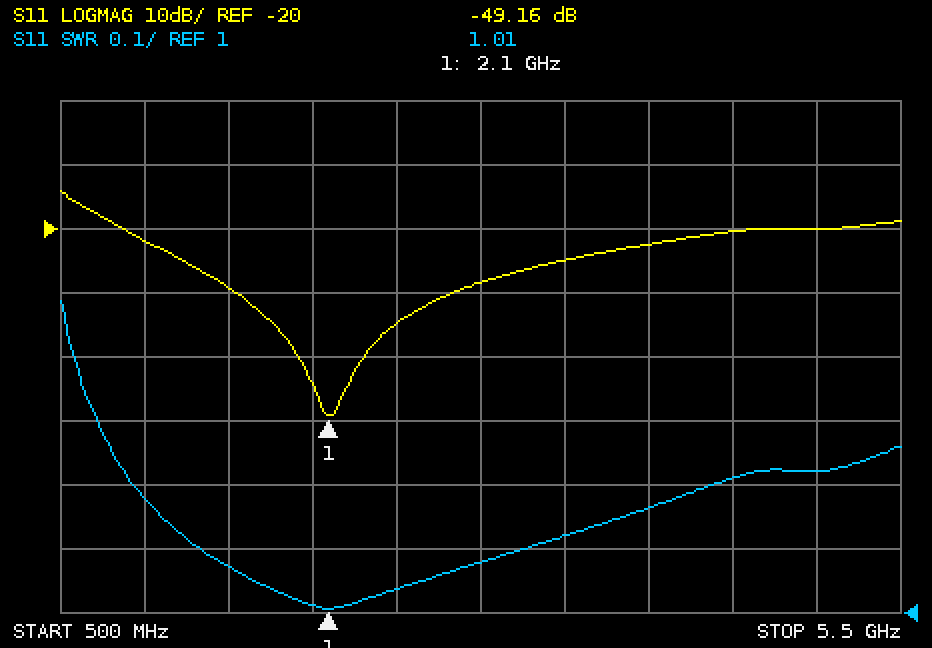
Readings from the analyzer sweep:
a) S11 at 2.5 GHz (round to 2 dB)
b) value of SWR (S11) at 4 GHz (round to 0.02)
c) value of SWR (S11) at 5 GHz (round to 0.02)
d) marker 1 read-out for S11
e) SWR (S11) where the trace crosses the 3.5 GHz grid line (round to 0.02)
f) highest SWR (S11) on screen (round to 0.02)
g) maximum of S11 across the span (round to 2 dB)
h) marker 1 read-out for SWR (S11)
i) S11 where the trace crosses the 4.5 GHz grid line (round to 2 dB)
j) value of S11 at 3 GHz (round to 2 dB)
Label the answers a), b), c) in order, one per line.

a) -34 dB
b) 1.16
c) 1.22
d) -49.16 dB
e) 1.12
f) 1.48
g) -14 dB
h) 1.01
i) -20 dB
j) -28 dB
